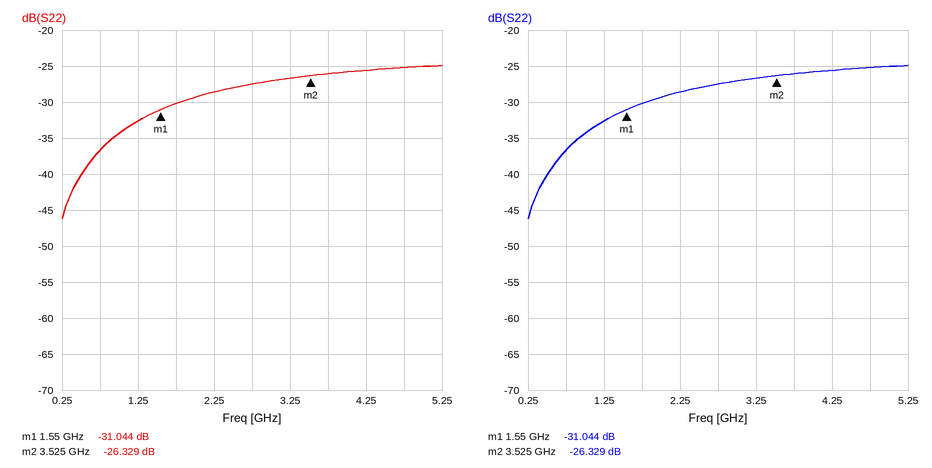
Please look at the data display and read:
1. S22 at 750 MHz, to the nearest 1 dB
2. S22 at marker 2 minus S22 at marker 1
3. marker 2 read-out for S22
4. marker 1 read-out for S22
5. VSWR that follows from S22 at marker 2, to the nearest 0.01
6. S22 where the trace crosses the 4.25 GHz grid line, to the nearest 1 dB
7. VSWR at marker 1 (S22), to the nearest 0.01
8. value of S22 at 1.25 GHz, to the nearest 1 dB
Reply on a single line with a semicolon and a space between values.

-37 dB; 4.715 dB; -26.329 dB; -31.044 dB; 1.10; -26 dB; 1.06; -33 dB
